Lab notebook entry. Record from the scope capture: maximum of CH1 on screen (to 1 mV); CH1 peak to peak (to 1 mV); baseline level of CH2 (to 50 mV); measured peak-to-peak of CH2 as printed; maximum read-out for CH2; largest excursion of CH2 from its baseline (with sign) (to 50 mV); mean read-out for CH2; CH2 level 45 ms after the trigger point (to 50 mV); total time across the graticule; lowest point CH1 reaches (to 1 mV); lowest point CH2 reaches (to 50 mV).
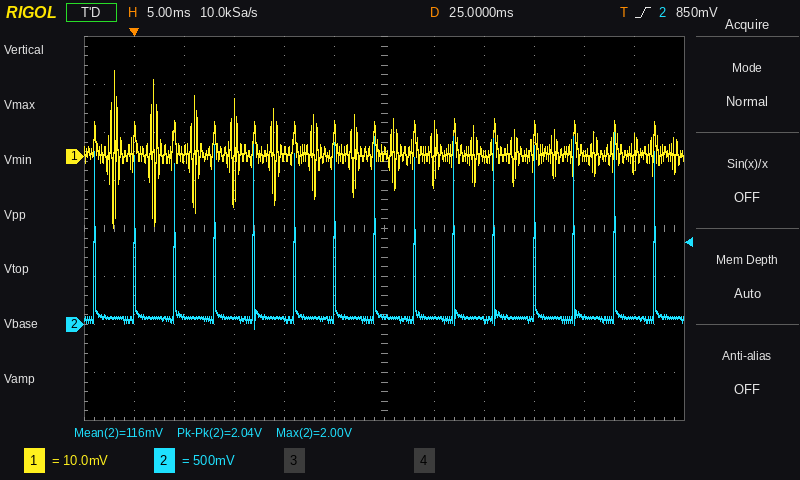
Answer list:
18 mV
33 mV
50 mV
2.04 V
2.00 V
+1.95 V
116 mV
100 mV
60 ms
-15 mV
-50 mV
